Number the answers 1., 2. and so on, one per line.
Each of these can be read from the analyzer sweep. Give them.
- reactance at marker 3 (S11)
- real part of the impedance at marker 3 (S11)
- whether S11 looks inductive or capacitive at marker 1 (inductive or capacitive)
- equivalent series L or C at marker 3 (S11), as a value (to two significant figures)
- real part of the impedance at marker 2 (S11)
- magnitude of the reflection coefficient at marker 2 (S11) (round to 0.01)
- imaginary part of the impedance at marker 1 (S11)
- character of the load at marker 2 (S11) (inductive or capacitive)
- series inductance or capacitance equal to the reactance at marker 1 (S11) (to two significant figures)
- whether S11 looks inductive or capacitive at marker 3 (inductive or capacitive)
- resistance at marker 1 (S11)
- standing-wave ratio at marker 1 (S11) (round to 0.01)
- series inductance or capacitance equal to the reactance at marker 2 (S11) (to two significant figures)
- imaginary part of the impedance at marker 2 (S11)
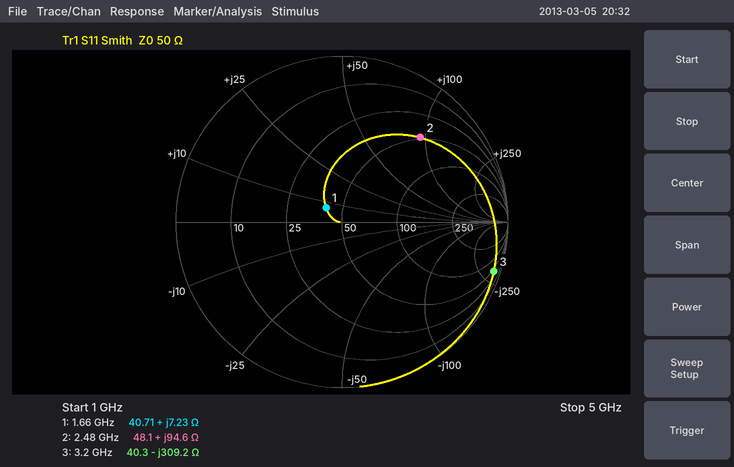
1. -309.2 Ω
2. 40.3 Ω
3. inductive
4. 160 fF
5. 48.1 Ω
6. 0.69
7. +7.23 Ω
8. inductive
9. 690 pH
10. capacitive
11. 40.71 Ω
12. 1.30
13. 6.1 nH
14. +94.6 Ω
